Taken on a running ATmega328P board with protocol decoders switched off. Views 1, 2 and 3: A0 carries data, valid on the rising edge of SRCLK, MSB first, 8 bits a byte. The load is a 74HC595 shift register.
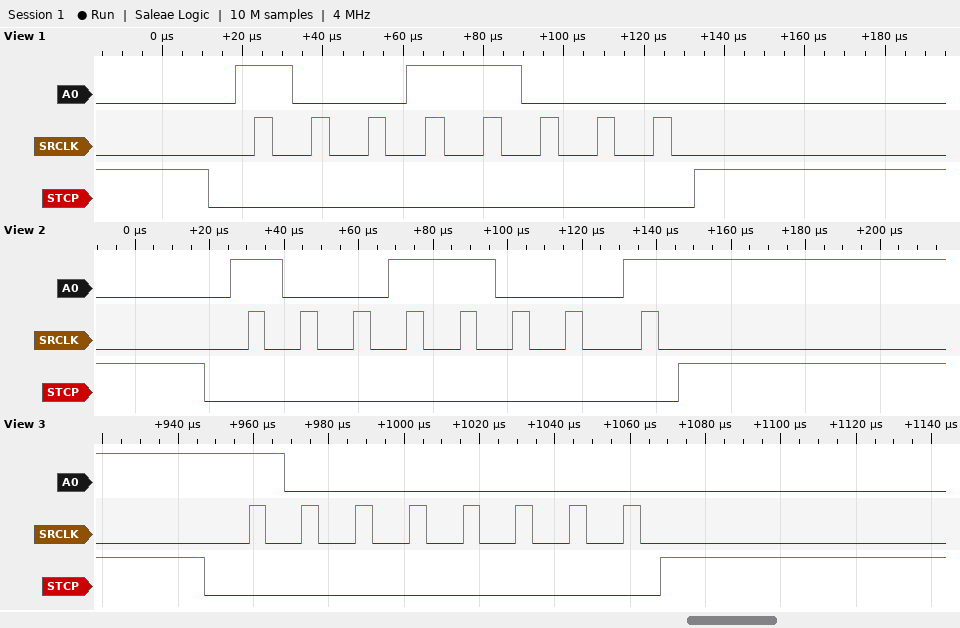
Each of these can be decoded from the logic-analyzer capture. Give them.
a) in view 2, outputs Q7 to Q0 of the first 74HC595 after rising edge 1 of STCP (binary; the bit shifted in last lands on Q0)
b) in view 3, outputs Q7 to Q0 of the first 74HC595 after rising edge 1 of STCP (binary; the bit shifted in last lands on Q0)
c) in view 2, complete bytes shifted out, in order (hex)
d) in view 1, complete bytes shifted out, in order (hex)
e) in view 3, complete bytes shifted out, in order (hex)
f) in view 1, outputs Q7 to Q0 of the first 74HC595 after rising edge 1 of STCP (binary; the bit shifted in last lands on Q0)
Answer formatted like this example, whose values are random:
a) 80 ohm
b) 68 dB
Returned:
a) 10011001
b) 10000000
c) 99
d) 0x98
e) 0x80
f) 10011000
